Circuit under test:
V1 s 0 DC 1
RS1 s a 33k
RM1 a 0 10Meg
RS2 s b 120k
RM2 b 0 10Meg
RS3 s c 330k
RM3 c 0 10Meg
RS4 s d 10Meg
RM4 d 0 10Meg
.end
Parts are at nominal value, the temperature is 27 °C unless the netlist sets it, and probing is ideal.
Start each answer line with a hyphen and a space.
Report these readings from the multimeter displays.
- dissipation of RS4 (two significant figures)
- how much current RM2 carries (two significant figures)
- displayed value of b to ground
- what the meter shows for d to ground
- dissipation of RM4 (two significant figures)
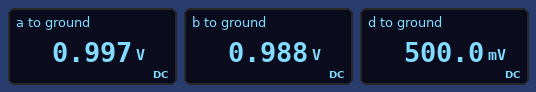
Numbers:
- 25 nW
- 99 nA
- 0.988 V
- 500.0 mV
- 25 nW
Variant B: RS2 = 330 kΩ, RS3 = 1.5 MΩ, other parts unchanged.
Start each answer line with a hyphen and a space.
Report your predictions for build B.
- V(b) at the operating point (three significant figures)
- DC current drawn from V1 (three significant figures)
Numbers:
- 968 mV
- 333 nA
